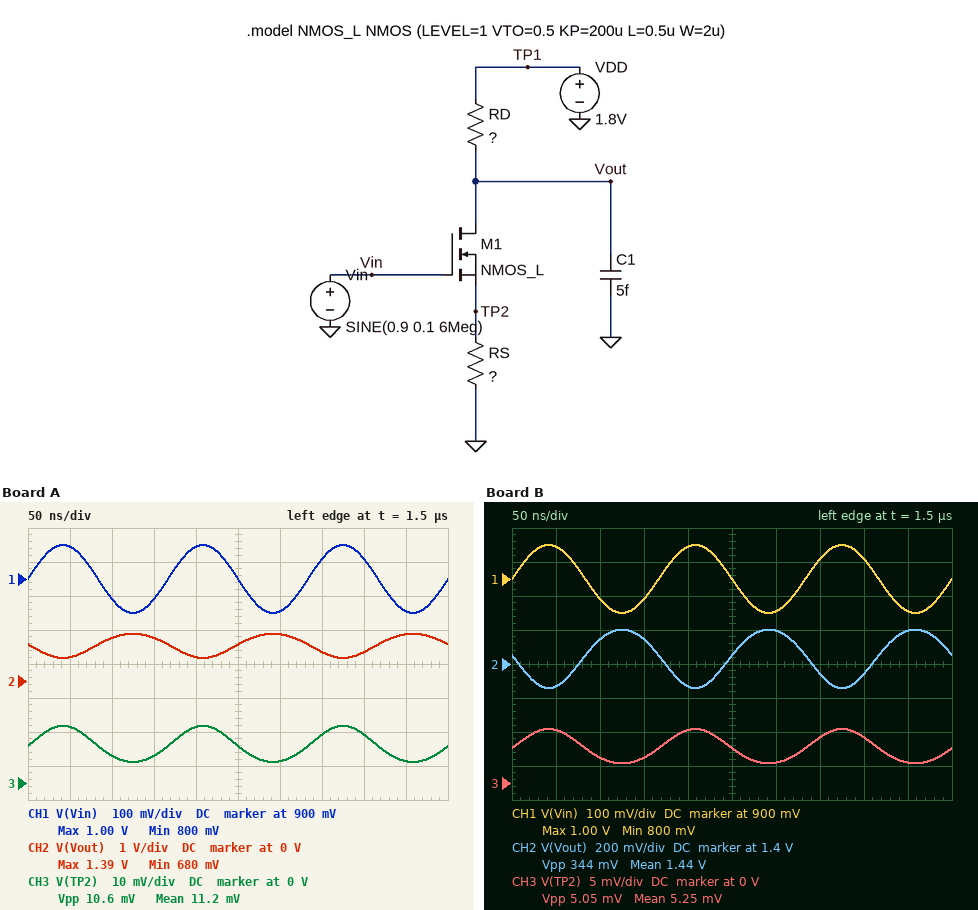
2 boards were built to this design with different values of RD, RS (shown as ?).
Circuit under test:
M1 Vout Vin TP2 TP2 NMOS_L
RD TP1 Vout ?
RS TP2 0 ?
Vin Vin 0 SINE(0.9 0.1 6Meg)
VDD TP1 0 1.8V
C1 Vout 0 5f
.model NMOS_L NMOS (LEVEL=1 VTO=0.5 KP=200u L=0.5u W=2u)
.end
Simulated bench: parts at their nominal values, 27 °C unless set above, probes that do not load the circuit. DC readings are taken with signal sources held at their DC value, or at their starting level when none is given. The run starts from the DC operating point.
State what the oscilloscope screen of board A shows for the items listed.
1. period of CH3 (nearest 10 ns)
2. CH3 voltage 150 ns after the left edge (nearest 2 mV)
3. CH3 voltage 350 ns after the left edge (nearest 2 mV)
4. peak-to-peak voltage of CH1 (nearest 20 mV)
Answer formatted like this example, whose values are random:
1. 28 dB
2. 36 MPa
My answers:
1. 170 ns
2. 8 mV
3. 14 mV
4. 200 mV
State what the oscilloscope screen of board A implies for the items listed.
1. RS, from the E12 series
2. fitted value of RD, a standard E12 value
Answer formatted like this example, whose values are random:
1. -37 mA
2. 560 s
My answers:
1. 180 Ω
2. 12 kΩ
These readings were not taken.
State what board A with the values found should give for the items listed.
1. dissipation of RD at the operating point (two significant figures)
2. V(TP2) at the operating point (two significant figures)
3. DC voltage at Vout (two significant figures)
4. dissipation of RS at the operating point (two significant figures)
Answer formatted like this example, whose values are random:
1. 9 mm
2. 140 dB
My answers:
1. 44 µW
2. 11 mV
3. 1.1 V
4. 660 nW
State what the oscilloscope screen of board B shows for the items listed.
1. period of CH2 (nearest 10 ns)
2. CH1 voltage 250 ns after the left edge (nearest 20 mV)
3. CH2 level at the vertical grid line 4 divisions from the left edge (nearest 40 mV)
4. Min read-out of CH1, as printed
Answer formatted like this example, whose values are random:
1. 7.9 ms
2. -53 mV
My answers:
1. 170 ns
2. 900 mV
3. 1.28 V
4. 800 mV
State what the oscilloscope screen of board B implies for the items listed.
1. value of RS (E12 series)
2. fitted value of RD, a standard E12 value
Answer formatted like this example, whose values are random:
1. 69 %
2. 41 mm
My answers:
1. 82 Ω
2. 5.6 kΩ
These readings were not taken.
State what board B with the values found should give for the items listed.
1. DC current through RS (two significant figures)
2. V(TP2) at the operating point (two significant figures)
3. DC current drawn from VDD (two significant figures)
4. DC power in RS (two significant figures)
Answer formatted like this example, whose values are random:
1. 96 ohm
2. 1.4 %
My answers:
1. 62 µA
2. 5.1 mV
3. 62 µA
4. 320 nW
